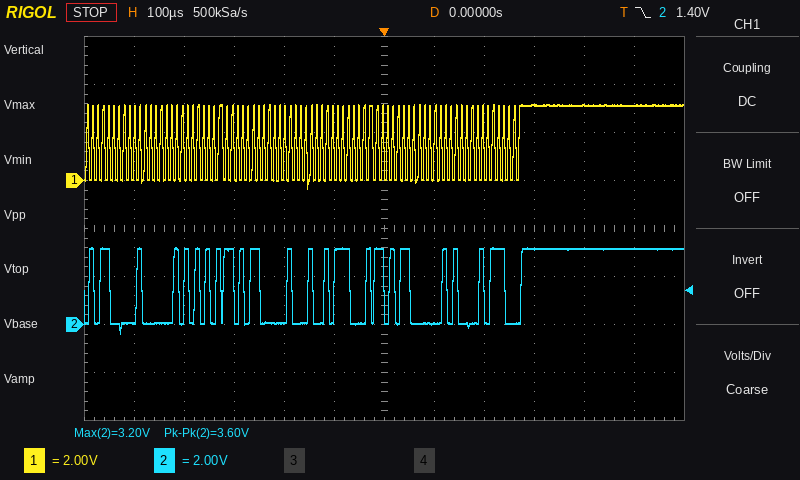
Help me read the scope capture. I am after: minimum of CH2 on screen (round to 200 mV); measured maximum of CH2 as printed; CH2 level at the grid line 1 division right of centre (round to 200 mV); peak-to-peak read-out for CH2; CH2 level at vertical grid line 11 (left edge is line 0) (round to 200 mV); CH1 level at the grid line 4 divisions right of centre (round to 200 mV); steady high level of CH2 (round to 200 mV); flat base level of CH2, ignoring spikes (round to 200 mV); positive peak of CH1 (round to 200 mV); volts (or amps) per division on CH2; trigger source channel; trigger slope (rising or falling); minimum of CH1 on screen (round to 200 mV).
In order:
-400 mV
3.20 V
0.0 V
3.60 V
3.2 V
3.2 V
3.2 V
0.0 V
3.2 V
2 V
CH2
falling
-400 mV
